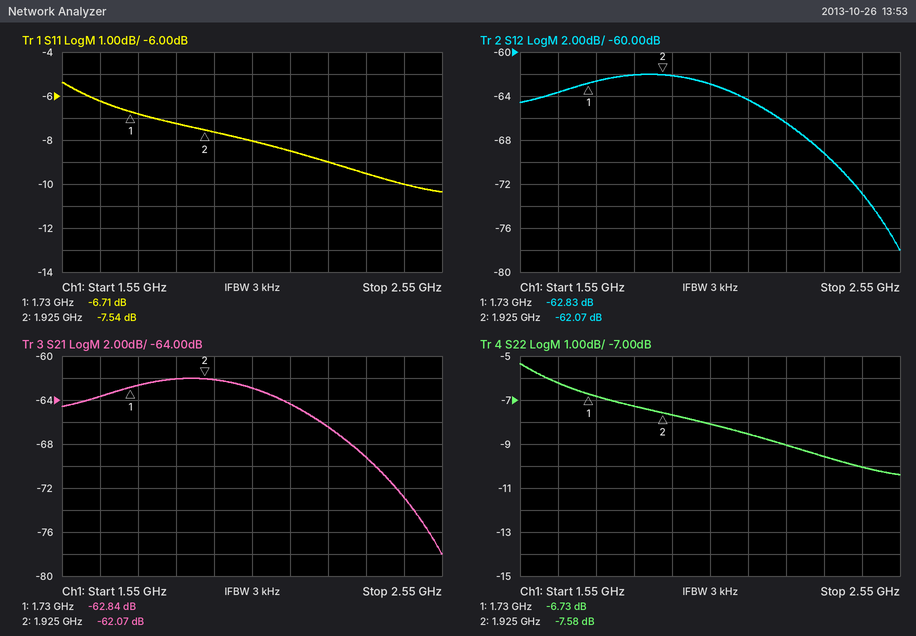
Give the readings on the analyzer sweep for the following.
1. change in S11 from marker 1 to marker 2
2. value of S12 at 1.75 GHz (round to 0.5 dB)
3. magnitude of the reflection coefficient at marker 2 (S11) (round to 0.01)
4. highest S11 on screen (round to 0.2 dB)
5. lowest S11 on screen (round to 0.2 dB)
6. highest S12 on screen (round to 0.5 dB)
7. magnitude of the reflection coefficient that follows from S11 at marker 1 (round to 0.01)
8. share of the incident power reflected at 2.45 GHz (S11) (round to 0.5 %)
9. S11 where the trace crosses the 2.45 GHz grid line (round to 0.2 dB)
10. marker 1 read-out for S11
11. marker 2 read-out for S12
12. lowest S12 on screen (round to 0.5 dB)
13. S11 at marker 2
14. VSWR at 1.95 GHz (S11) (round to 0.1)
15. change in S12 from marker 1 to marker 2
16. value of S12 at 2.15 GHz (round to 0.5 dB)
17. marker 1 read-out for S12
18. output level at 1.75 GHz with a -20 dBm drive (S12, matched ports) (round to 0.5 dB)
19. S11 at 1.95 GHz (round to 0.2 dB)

-0.83 dB
-62.5 dB
0.42
-5.4 dB
-10.4 dB
-62.0 dB
0.46
10.0 %
-10.0 dB
-6.71 dB
-62.07 dB
-78.0 dB
-7.54 dB
2.4
0.76 dB
-64.5 dB
-62.83 dB
-82.5 dBm
-7.6 dB
